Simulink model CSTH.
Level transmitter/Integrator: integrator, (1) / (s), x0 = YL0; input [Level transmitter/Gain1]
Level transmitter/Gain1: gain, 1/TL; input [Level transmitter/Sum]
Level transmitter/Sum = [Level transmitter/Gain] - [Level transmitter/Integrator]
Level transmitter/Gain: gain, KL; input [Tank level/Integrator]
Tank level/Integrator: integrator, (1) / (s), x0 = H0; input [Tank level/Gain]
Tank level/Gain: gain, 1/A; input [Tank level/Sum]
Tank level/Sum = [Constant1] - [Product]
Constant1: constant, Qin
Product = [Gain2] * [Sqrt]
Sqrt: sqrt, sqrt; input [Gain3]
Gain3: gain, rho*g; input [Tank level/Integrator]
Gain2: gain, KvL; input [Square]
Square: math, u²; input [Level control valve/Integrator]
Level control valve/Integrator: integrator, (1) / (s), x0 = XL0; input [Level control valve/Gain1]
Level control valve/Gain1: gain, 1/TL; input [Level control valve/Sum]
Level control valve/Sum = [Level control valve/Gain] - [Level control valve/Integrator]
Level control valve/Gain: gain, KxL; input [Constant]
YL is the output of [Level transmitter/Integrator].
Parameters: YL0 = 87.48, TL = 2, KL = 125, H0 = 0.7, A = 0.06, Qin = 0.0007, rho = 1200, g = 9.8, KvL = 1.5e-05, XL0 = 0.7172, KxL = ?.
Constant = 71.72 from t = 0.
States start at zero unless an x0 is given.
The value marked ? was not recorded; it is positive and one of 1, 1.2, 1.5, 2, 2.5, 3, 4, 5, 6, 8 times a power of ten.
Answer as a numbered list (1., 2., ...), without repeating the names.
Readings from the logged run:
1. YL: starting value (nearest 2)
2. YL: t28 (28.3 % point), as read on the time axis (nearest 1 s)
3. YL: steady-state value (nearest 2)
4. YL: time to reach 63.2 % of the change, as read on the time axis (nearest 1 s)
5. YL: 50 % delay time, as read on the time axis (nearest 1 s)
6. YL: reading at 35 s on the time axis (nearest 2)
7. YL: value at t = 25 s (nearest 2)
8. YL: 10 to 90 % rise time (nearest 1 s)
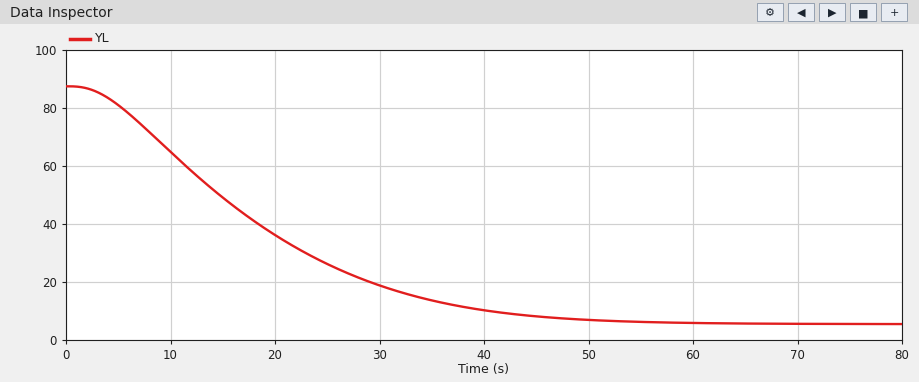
1. 88
2. 10 s
3. 6
4. 20 s
5. 16 s
6. 14
7. 26
8. 29 s
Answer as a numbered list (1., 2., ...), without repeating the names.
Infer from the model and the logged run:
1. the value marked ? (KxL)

1. 0.02
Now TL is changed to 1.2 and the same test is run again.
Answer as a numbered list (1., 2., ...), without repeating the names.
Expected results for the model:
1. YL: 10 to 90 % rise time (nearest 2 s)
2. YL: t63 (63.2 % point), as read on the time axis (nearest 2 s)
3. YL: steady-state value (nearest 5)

1. 28 s
2. 18 s
3. 5
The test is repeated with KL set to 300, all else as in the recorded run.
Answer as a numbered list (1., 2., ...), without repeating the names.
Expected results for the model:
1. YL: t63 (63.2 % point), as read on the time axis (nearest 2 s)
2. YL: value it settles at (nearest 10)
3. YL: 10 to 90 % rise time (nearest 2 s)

1. 32 s
2. 10
3. 22 s
